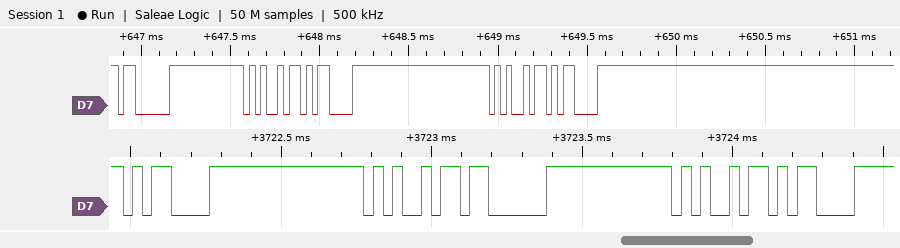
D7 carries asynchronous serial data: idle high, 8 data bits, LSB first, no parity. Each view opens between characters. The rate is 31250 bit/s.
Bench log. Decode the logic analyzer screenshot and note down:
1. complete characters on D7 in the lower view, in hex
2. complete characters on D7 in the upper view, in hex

0D, A5, 03, A5, 0D
03, A5, 0D, A5, 0D
